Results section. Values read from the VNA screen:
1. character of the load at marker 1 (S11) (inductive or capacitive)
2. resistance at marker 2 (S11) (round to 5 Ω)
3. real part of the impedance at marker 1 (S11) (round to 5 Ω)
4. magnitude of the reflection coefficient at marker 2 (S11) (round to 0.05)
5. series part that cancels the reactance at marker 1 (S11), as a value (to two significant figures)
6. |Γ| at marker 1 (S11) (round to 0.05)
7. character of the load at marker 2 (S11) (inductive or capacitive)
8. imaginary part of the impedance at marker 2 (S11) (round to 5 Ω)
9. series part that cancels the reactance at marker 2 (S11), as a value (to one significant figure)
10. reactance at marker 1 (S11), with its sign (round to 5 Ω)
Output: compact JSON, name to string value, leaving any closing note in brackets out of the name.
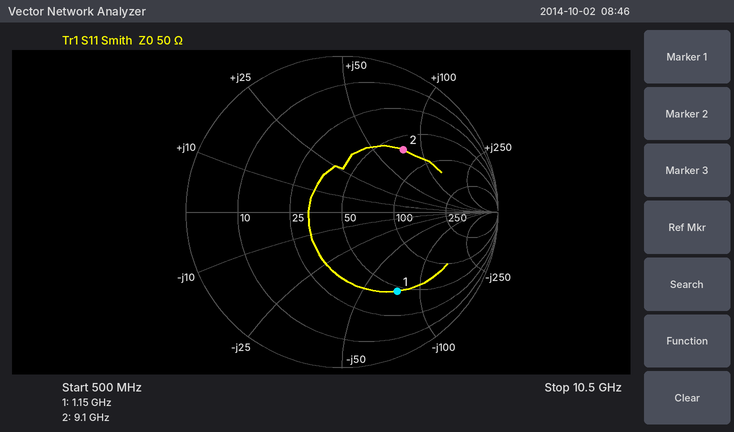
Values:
{"character of the load at marker 1 (S11)": "capacitive", "resistance at marker 2 (S11)": "65 Ω", "real part of the impedance at marker 1 (S11)": "45 Ω", "magnitude of the reflection coefficient at marker 2 (S11)": "0.55", "series part that cancels the reactance at marker 1 (S11), as a value": "10 nH", "|Γ| at marker 1 (S11)": "0.60", "character of the load at marker 2 (S11)": "inductive", "imaginary part of the impedance at marker 2 (S11)": "+75 Ω", "series part that cancels the reactance at marker 2 (S11), as a value": "200 fF", "reactance at marker 1 (S11), with its sign": "-75 Ω"}
